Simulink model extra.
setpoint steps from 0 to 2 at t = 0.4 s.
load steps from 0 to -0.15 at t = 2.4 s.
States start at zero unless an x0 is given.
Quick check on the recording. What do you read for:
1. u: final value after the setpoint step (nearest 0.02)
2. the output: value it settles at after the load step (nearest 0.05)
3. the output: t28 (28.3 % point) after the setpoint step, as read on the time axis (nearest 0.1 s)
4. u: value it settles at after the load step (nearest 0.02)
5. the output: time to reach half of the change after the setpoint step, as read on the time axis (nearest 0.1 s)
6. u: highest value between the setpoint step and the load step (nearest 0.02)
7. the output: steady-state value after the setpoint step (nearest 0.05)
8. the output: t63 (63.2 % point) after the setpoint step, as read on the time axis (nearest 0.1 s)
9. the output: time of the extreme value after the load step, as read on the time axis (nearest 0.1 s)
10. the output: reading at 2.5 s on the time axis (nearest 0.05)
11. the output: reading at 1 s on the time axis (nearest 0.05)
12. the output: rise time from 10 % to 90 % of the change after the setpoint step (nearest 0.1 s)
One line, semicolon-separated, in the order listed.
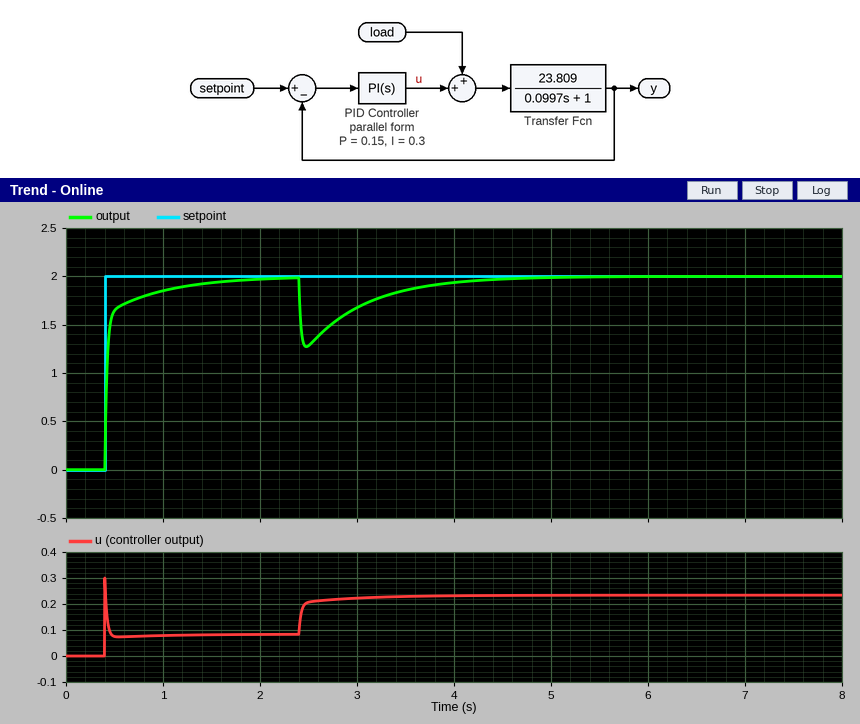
0.08; 2.00; 0.4 s; 0.24; 0.4 s; 0.30; 2.00; 0.4 s; 2.5 s; 1.30; 1.85; 0.4 s
